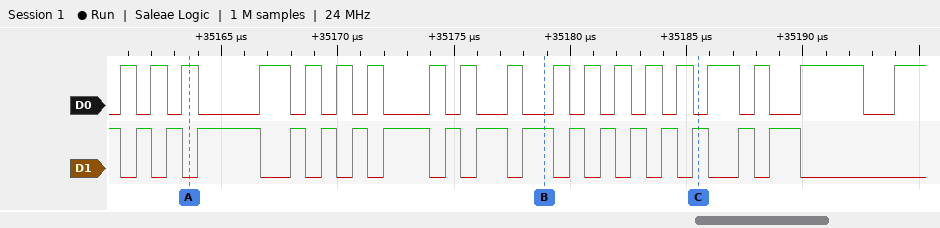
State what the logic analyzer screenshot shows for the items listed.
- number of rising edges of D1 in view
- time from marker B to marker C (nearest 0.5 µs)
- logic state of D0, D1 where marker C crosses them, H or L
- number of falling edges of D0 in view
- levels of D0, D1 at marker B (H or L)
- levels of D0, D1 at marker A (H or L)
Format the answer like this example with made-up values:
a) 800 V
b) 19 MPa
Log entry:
a) 17
b) 6.5 µs
c) D0=L, D1=H
d) 18
e) D0=L, D1=H
f) D0=H, D1=L
